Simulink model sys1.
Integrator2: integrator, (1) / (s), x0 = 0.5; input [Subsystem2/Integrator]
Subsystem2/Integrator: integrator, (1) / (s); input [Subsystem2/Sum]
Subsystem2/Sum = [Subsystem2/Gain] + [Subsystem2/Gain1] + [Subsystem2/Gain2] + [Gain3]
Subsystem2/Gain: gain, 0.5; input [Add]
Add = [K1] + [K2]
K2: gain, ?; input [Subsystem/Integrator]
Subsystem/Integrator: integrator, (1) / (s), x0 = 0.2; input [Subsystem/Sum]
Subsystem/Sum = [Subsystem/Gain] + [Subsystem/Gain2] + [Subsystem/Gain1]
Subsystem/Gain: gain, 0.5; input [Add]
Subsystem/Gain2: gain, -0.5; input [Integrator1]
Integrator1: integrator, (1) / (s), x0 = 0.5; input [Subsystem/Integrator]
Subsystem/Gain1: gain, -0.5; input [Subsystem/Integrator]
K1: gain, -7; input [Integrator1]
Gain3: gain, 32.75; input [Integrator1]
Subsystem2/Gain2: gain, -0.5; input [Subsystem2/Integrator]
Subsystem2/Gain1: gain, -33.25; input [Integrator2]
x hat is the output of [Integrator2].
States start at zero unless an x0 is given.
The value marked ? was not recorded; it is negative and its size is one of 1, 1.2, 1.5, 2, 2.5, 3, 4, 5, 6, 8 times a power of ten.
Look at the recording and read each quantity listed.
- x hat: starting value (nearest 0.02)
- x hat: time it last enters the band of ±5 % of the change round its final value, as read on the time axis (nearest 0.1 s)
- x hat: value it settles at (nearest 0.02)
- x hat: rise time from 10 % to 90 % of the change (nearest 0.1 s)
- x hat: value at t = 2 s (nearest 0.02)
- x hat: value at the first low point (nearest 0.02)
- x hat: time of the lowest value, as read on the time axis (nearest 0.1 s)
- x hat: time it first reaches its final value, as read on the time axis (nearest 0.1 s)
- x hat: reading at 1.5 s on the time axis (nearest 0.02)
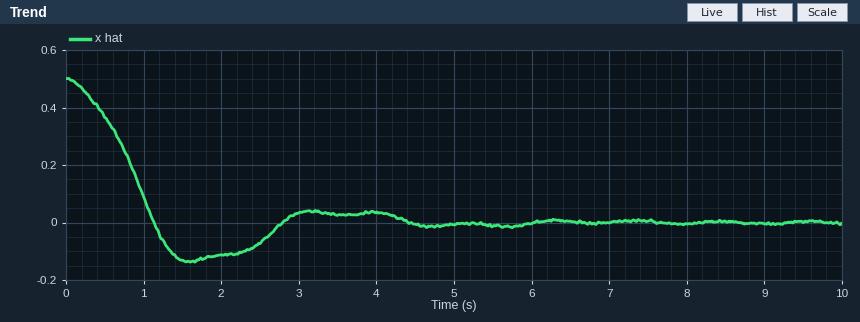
0.50
4.2 s
0.00
0.8 s
-0.12
-0.14
1.6 s
1.1 s
-0.14
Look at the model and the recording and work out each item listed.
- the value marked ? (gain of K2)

-2
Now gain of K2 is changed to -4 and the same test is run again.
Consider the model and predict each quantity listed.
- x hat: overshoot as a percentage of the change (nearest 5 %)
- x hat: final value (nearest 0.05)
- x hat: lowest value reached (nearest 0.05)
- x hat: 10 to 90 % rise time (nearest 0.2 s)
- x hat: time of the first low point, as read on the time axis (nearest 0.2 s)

10 %
0.00
-0.05
1.0 s
2.4 s
